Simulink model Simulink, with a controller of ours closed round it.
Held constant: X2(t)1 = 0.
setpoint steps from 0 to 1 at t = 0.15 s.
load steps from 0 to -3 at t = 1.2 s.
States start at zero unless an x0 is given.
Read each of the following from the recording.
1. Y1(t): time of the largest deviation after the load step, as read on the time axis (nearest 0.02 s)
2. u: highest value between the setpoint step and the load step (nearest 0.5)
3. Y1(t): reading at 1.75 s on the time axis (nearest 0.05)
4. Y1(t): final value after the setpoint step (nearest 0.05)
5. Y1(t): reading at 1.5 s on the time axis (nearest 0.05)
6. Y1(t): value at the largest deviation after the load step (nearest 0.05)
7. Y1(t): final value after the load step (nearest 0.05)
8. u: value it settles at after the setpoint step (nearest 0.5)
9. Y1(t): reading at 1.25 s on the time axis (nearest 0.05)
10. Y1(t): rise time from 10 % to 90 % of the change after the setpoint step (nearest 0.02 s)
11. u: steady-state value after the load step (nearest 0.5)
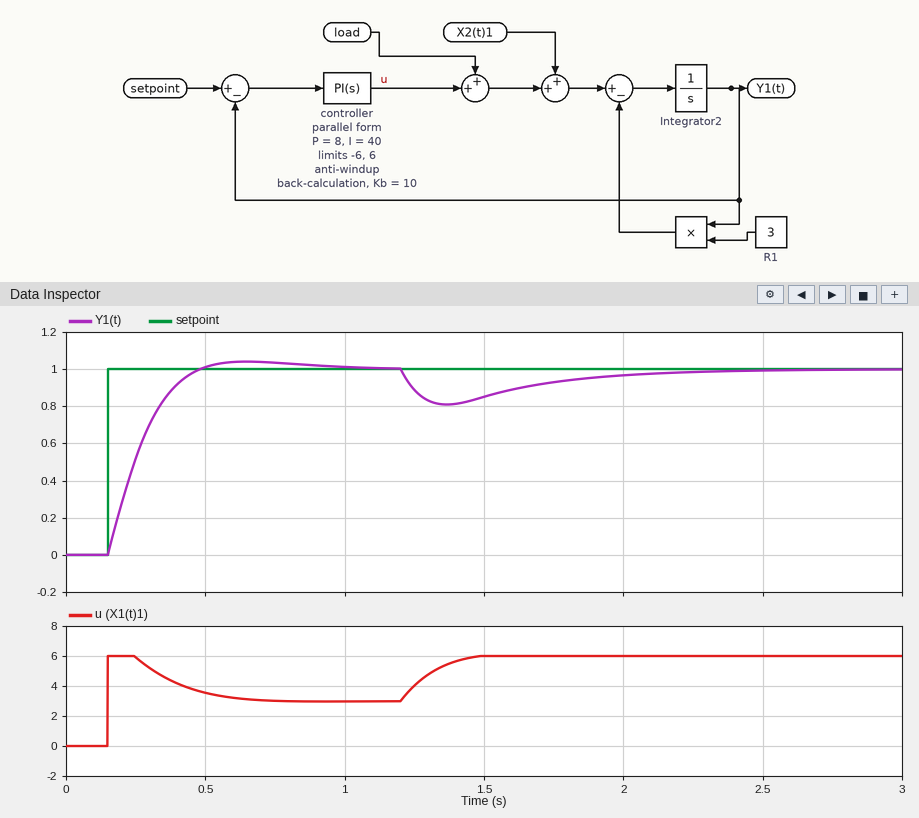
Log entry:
1.36 s
6.0
0.95
1.00
0.85
0.80
1.00
3.0
0.90
0.22 s
6.0
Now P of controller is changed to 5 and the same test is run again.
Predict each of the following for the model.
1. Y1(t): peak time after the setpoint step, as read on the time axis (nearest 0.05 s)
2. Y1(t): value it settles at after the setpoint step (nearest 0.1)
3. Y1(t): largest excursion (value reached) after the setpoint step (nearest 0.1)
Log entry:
0.60 s
1.0
1.1
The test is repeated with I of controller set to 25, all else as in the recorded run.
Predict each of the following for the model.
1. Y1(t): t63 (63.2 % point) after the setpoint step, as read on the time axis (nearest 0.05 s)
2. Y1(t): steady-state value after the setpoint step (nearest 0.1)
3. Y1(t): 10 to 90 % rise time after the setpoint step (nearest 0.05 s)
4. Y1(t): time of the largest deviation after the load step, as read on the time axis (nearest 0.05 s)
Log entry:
0.30 s
1.0
0.30 s
1.40 s
